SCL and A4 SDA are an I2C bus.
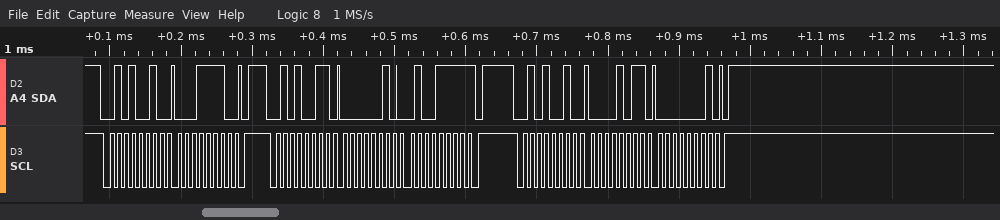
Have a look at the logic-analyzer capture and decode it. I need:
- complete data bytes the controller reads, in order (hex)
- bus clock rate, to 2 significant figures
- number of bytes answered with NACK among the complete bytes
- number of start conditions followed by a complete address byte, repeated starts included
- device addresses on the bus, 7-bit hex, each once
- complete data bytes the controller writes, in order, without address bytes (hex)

02 4F
100 kHz
1
3
0x29
1E 0B 01
